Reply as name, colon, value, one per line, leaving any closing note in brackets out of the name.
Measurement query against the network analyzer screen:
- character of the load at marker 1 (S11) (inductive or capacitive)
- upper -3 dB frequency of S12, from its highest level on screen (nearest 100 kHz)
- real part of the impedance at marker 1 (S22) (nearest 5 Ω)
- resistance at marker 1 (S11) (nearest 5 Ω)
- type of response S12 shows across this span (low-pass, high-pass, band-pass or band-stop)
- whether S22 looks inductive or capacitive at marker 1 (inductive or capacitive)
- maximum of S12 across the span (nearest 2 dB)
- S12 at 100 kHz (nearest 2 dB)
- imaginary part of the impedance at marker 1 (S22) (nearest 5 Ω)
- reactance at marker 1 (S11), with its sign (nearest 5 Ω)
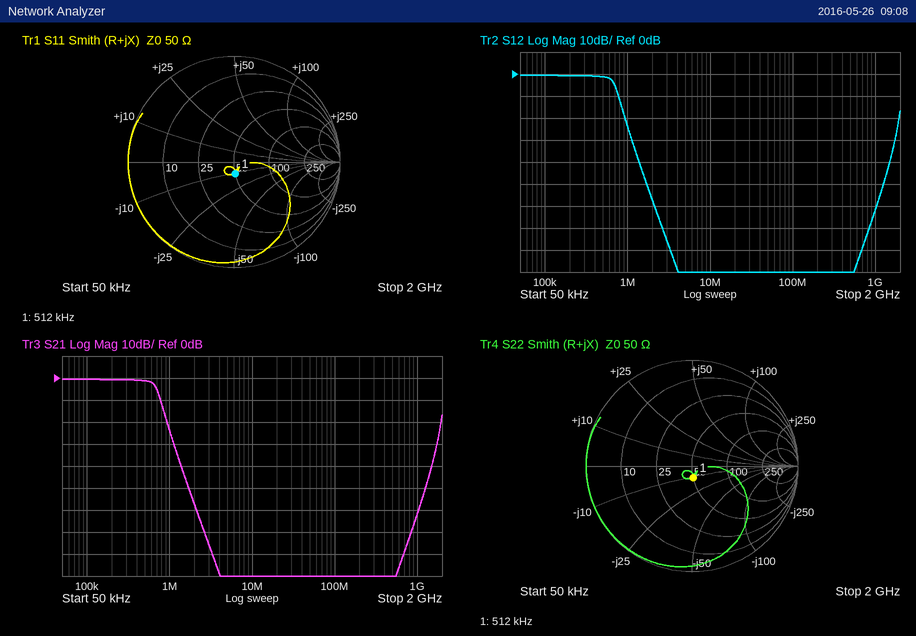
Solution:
character of the load at marker 1 (S11): capacitive
upper -3 dB frequency of S12, from its highest level on screen: 700 kHz
real part of the impedance at marker 1 (S22): 50 Ω
resistance at marker 1 (S11): 50 Ω
type of response S12 shows across this span: low-pass
whether S22 looks inductive or capacitive at marker 1: capacitive
maximum of S12 across the span: 0 dB
S12 at 100 kHz: 0 dB
imaginary part of the impedance at marker 1 (S22): -10 Ω
reactance at marker 1 (S11), with its sign: -10 Ω
